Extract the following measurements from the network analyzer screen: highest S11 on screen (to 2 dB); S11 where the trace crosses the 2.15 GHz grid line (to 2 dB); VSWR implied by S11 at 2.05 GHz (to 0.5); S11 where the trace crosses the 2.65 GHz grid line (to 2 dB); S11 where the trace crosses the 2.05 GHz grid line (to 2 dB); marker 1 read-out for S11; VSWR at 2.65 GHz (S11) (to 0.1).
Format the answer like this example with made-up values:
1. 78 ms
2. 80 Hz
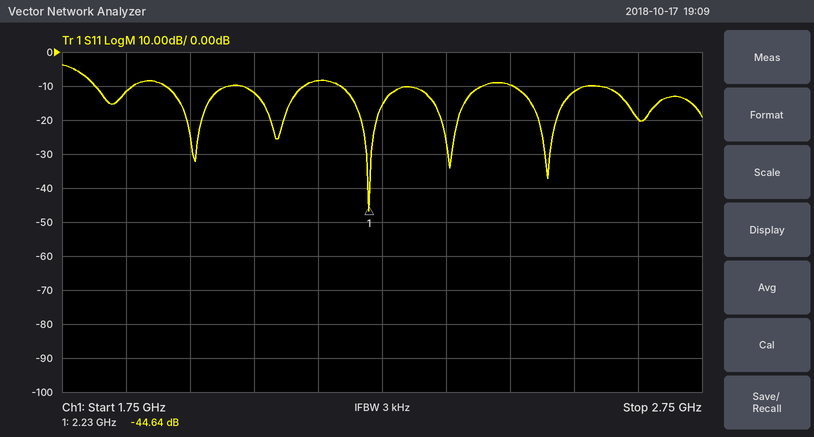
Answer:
1. -4 dB
2. -8 dB
3. 1.5
4. -20 dB
5. -12 dB
6. -44.64 dB
7. 1.2
